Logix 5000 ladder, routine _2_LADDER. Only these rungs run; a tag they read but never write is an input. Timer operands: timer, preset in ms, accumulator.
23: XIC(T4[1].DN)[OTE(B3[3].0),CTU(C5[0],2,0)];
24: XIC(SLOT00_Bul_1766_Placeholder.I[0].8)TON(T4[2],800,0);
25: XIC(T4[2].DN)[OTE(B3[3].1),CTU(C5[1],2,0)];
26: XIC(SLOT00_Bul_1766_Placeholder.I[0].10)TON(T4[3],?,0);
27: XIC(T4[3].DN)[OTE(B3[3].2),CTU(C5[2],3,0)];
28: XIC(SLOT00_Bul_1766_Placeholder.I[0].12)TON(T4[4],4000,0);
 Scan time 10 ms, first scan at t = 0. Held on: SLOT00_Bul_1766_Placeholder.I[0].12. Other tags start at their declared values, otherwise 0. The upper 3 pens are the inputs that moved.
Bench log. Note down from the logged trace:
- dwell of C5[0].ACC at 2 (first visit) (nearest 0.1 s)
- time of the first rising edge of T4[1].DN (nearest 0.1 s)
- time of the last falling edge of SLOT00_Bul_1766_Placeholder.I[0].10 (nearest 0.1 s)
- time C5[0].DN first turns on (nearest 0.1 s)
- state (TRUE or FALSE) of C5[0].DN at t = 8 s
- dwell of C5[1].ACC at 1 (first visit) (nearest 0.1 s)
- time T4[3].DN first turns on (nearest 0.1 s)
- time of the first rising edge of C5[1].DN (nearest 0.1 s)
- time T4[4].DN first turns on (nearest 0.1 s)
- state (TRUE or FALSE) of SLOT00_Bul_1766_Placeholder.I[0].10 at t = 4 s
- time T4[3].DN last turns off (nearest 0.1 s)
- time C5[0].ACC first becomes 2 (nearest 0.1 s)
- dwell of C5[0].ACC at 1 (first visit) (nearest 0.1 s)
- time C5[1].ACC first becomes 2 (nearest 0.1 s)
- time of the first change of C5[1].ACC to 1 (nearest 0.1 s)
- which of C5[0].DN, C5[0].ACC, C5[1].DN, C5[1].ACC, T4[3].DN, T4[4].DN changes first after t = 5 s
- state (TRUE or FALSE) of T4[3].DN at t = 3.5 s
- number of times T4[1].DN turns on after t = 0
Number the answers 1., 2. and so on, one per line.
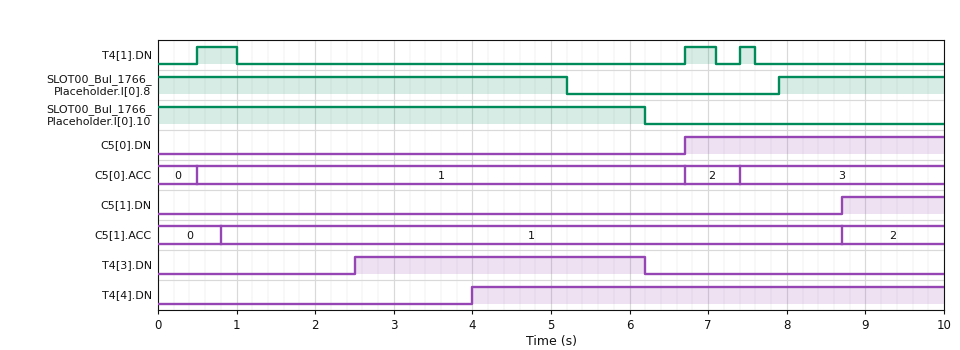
1. 0.7 s
2. 0.5 s
3. 6.2 s
4. 6.7 s
5. TRUE
6. 7.9 s
7. 2.5 s
8. 8.7 s
9. 4.0 s
10. TRUE
11. 6.2 s
12. 6.7 s
13. 6.2 s
14. 8.7 s
15. 0.8 s
16. T4[3].DN
17. TRUE
18. 3
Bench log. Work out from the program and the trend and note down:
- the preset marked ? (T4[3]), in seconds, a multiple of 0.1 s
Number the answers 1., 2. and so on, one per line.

1. 2.5 s
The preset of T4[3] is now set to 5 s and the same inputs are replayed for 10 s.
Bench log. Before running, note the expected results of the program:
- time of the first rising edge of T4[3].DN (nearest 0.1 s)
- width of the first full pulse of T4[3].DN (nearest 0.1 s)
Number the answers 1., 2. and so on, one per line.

1. 5.0 s
2. 1.2 s
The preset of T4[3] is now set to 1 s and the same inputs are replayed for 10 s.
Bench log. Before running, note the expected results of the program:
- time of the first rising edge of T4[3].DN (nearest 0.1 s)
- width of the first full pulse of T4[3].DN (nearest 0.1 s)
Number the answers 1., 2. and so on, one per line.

1. 1.0 s
2. 5.2 s
